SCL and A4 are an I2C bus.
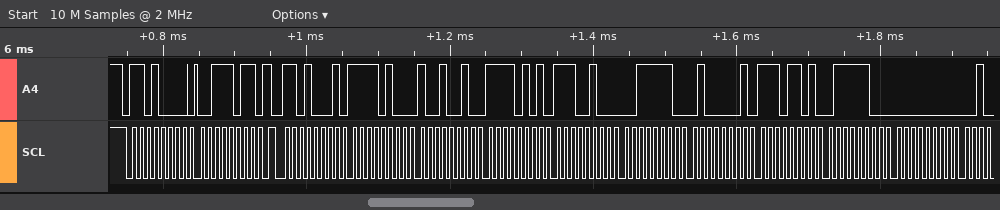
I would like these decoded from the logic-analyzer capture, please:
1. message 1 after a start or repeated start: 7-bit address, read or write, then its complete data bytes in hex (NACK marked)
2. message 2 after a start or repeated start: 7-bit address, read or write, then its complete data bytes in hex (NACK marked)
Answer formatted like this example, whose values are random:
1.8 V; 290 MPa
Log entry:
0x68 write: 3B; 0x68 read: F4 92 F5 E4 3E 41 ED 7C 00
